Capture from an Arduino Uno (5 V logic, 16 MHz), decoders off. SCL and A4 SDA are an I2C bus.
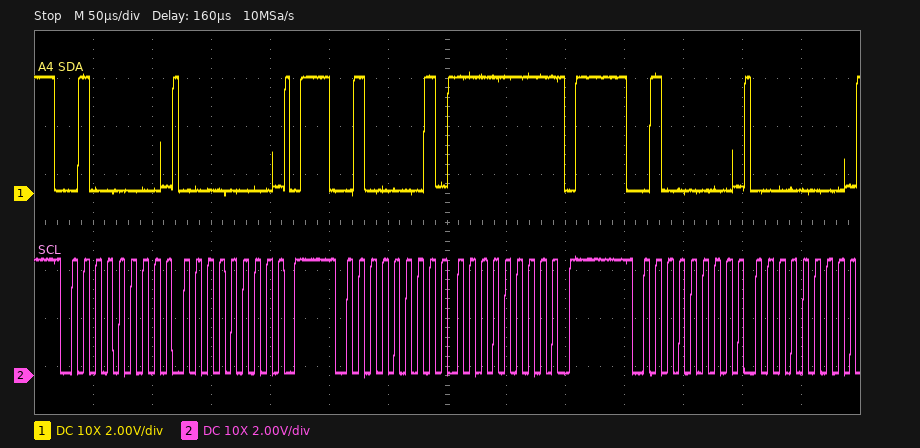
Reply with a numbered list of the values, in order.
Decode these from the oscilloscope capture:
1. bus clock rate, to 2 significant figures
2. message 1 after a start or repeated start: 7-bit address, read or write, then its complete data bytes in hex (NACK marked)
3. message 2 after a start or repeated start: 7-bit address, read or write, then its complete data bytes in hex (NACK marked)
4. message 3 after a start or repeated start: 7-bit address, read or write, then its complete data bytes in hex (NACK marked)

1. 100 kHz
2. 0x20 write: 00
3. 0x20 read: FF NACK
4. 0x20 write: 00
